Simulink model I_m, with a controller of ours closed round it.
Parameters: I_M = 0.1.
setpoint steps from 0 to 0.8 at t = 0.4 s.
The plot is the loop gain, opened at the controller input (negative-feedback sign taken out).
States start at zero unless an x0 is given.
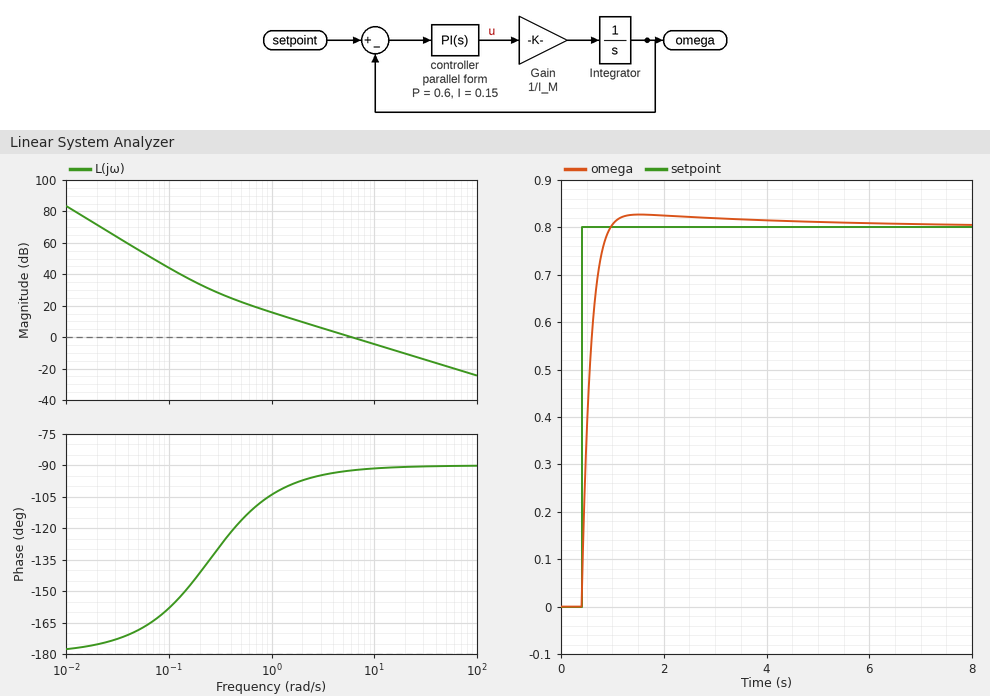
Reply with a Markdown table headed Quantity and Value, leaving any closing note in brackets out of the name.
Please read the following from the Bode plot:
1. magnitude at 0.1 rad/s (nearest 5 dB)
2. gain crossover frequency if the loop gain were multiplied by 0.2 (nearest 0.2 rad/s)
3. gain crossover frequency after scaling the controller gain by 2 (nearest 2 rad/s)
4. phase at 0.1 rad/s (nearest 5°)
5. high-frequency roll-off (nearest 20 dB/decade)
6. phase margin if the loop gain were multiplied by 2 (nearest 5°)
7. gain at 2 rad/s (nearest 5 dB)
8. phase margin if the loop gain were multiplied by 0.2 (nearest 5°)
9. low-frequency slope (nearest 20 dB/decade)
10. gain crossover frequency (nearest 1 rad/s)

| Quantity | Value |
|---|---|
| magnitude at 0.1 rad/s | 45 dB |
| gain crossover frequency if the loop gain were multiplied by 0.2 | 1.2 rad/s |
| gain crossover frequency after scaling the controller gain by 2 | 12 rad/s |
| phase at 0.1 rad/s | -160° |
| high-frequency roll-off | -20 dB/decade |
| phase margin if the loop gain were multiplied by 2 | 90° |
| gain at 2 rad/s | 10 dB |
| phase margin if the loop gain were multiplied by 0.2 | 80° |
| low-frequency slope | -40 dB/decade |
| gain crossover frequency | 6 rad/s |
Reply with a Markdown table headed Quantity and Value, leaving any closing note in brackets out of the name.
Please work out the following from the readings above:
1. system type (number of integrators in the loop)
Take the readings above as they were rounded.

| Quantity | Value |
|---|---|
| system type | 2 |
